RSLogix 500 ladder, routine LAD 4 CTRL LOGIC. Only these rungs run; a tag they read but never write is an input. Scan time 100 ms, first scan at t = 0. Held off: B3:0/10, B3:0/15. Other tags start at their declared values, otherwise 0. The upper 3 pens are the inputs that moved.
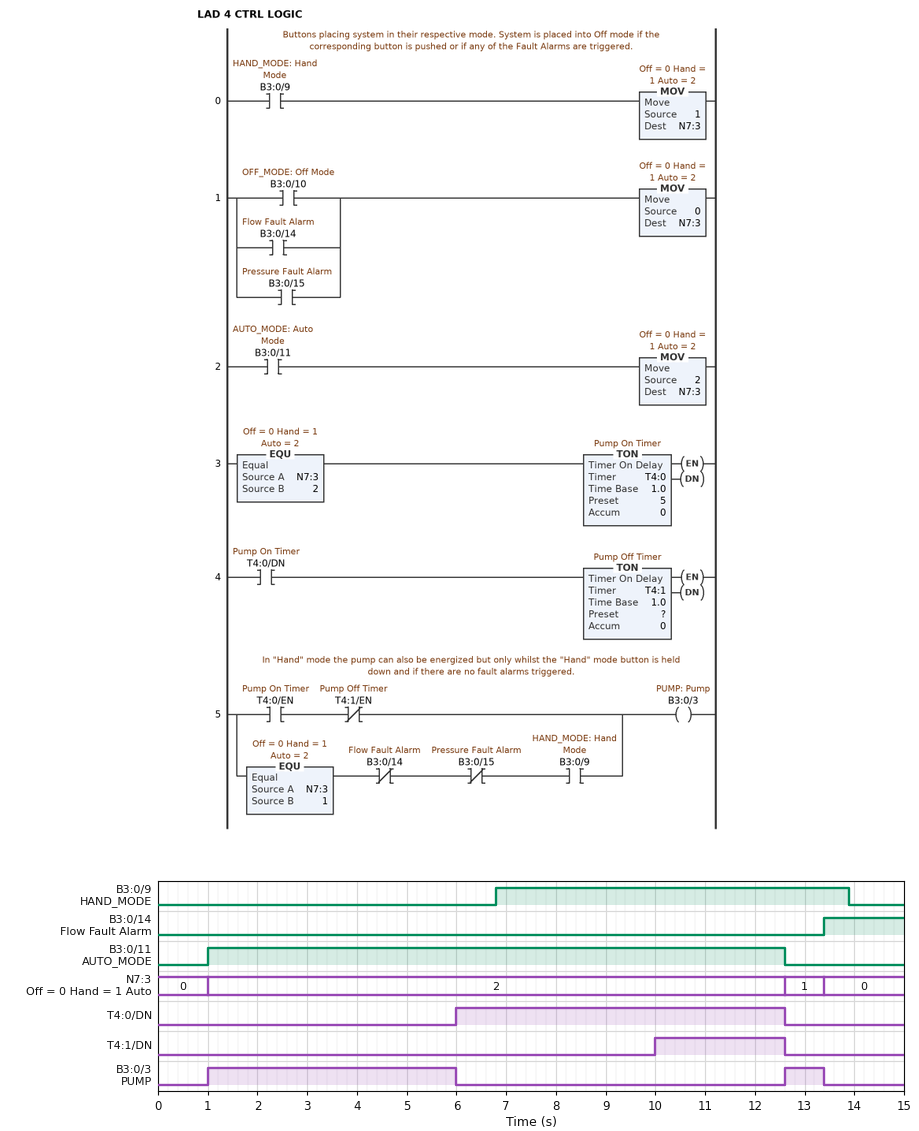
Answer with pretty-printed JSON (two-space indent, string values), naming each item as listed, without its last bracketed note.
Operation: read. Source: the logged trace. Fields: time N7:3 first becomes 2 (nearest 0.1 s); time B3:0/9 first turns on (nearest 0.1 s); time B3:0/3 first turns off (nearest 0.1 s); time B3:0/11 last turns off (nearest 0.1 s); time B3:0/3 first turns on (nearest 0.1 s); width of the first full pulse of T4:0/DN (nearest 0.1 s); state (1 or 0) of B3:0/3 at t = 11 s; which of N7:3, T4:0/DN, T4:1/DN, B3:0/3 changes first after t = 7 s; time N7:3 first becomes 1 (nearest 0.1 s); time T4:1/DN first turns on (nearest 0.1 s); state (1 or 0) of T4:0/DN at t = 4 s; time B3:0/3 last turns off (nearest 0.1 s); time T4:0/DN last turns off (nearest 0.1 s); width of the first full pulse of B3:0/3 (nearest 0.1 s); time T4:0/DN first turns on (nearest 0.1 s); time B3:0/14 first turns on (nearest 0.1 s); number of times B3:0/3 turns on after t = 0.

{
  "time N7:3 first becomes 2": "1.0 s",
  "time B3:0/9 first turns on": "6.8 s",
  "time B3:0/3 first turns off": "6.0 s",
  "time B3:0/11 last turns off": "12.6 s",
  "time B3:0/3 first turns on": "1.0 s",
  "width of the first full pulse of T4:0/DN": "6.6 s",
  "state (1 or 0) of B3:0/3 at t = 11 s": "0",
  "which of N7:3, T4:0/DN, T4:1/DN, B3:0/3 changes first after t = 7 s": "T4:1/DN",
  "time N7:3 first becomes 1": "12.6 s",
  "time T4:1/DN first turns on": "10.0 s",
  "state (1 or 0) of T4:0/DN at t = 4 s": "0",
  "time B3:0/3 last turns off": "13.4 s",
  "time T4:0/DN last turns off": "12.6 s",
  "width of the first full pulse of B3:0/3": "5.0 s",
  "time T4:0/DN first turns on": "6.0 s",
  "time B3:0/14 first turns on": "13.4 s",
  "number of times B3:0/3 turns on after t = 0": "2"
}
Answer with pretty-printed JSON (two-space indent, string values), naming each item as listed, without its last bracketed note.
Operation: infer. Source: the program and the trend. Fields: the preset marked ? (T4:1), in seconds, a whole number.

{
  "the preset marked ? (T4:1), in seconds, a whole number": "4 s"
}
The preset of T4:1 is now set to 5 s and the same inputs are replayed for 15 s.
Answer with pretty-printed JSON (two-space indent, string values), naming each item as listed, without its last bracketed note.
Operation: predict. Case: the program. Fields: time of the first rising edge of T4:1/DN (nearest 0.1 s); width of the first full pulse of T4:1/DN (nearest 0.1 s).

{
  "time of the first rising edge of T4:1/DN": "11.0 s",
  "width of the first full pulse of T4:1/DN": "1.6 s"
}
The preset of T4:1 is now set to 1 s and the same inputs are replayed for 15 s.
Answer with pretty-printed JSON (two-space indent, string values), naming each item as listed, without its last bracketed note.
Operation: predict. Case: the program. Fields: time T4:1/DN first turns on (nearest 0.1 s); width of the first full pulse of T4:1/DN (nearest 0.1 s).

{
  "time T4:1/DN first turns on": "7.0 s",
  "width of the first full pulse of T4:1/DN": "5.6 s"
}
